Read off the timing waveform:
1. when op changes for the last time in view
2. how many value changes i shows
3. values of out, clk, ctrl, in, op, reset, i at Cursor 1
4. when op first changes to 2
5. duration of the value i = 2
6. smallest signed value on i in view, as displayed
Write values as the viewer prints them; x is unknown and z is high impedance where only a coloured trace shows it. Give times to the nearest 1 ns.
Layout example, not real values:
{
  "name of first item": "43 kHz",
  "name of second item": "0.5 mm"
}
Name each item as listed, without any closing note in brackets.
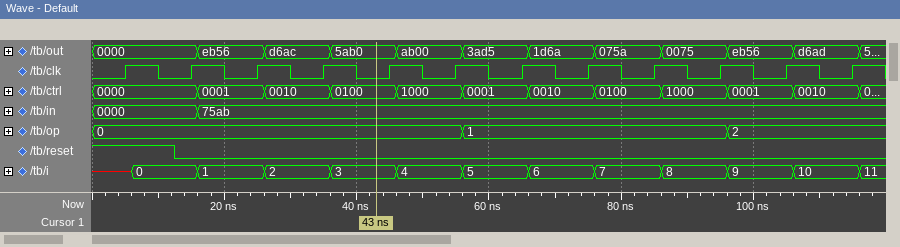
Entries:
{
  "when op changes for the last time in view": "96 ns",
  "how many value changes i shows": "12",
  "values of out, clk, ctrl, in, op, reset, i at Cursor 1": "out=5ab0, clk=0, ctrl=0100, in=75ab, op=0, reset=0, i=3",
  "when op first changes to 2": "96 ns",
  "duration of the value i = 2": "10 ns",
  "smallest signed value on i in view, as displayed": "0"
}
